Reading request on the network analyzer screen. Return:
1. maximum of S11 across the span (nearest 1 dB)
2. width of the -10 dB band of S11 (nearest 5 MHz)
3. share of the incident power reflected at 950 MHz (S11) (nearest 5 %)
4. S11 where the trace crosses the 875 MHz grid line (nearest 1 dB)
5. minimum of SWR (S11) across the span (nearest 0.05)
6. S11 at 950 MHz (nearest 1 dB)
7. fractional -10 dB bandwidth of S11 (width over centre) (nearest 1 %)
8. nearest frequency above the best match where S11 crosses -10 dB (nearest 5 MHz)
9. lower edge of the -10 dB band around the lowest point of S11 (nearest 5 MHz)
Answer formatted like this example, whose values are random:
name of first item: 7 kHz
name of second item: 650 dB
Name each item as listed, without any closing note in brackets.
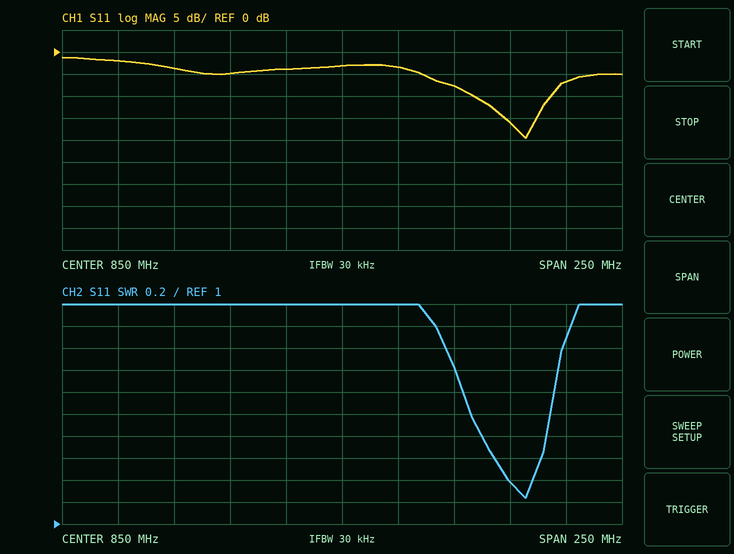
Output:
maximum of S11 across the span: -1 dB
width of the -10 dB band of S11: 35 MHz
share of the incident power reflected at 950 MHz (S11): 20 %
S11 where the trace crosses the 875 MHz grid line: -3 dB
minimum of SWR (S11) across the span: 1.25
S11 at 950 MHz: -7 dB
fractional -10 dB bandwidth of S11 (width over centre): 4 %
nearest frequency above the best match where S11 crosses -10 dB: 945 MHz
lower edge of the -10 dB band around the lowest point of S11: 910 MHz
